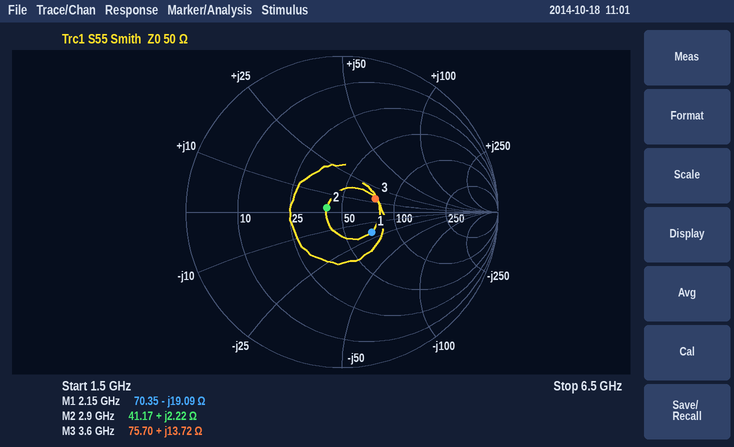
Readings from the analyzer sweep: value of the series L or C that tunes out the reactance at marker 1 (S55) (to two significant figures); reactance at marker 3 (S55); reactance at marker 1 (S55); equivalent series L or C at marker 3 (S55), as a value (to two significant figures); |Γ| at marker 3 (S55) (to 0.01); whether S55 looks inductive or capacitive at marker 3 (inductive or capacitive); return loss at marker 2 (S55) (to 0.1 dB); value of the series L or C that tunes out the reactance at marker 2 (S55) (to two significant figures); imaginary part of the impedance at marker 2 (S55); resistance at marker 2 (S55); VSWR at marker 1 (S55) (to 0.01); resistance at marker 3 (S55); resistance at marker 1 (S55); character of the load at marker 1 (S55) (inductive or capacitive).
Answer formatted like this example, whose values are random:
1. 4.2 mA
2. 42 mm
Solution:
1. 1.4 nH
2. +13.72 Ω
3. -19.09 Ω
4. 610 pH
5. 0.23
6. inductive
7. 20.0 dB
8. 25 pF
9. +2.22 Ω
10. 41.17 Ω
11. 1.59
12. 75.70 Ω
13. 70.35 Ω
14. capacitive
